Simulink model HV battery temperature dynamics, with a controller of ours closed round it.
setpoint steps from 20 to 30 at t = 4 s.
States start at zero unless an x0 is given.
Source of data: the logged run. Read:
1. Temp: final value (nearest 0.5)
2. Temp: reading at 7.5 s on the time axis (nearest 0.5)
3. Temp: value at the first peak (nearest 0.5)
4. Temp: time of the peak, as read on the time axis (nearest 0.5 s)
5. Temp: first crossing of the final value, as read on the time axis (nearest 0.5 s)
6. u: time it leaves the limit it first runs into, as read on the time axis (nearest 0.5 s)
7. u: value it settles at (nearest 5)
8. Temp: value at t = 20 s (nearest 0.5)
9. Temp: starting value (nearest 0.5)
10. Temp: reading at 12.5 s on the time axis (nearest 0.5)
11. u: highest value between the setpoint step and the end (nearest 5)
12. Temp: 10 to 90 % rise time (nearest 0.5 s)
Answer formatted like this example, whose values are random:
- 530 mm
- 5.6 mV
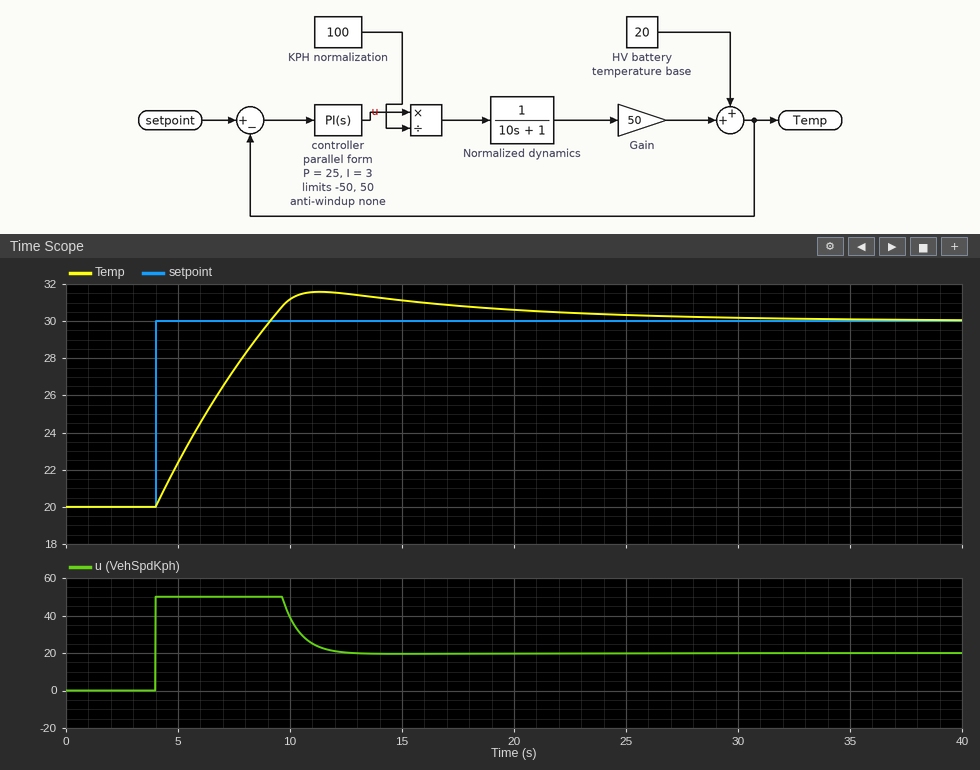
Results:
- 30.0
- 27.5
- 31.5
- 11.5 s
- 9.0 s
- 9.5 s
- 20
- 30.5
- 20.0
- 31.5
- 50
- 4.0 s
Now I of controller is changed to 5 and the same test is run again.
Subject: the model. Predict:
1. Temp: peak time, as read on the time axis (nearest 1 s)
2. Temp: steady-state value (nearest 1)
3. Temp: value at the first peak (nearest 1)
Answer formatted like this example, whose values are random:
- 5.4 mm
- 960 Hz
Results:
- 12 s
- 30
- 33
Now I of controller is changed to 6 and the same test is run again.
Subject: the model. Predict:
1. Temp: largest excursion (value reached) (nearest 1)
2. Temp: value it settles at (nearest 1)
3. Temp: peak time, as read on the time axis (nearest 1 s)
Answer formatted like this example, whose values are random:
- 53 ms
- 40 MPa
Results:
- 33
- 30
- 12 s
